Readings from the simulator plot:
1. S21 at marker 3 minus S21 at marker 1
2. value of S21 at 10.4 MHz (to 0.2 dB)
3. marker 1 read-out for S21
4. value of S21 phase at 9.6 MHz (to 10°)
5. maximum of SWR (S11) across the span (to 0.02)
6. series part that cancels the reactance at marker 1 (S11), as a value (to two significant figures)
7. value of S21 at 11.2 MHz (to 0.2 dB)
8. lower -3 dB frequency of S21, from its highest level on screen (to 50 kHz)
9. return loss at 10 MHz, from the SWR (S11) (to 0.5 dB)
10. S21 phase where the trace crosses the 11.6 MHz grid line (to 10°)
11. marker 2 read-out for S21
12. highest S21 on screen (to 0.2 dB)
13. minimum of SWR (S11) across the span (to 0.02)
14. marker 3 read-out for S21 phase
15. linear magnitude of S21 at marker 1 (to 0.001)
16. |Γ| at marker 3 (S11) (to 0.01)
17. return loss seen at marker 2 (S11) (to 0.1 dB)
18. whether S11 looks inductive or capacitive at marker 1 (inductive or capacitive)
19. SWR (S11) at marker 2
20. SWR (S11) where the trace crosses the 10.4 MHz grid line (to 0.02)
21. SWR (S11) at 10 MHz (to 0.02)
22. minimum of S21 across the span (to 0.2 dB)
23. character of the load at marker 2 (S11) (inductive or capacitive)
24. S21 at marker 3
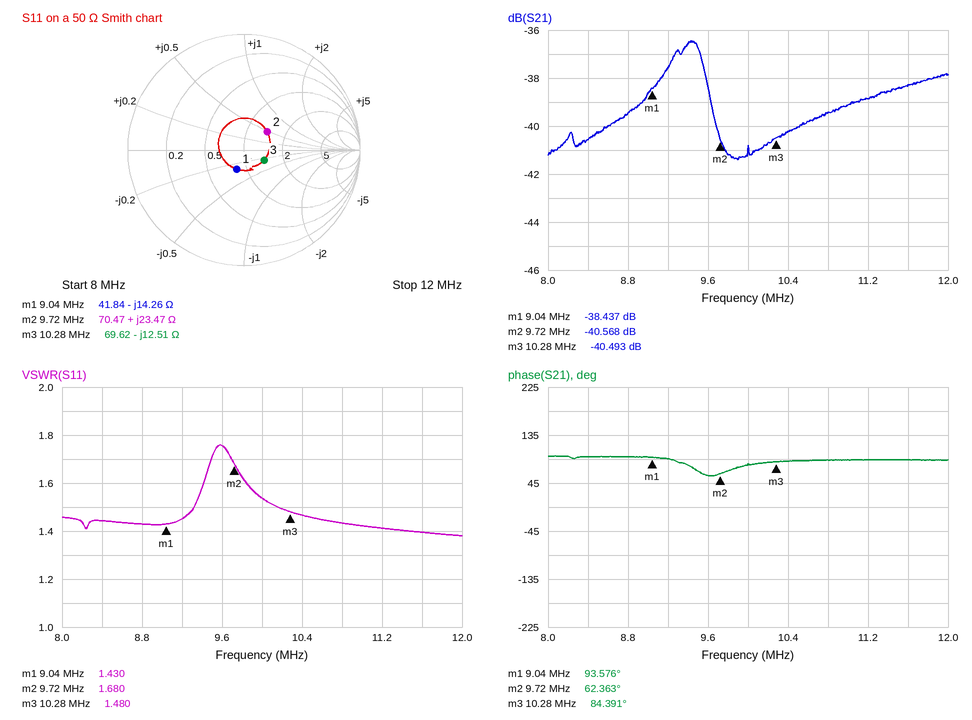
-2.056 dB
-40.2 dB
-38.437 dB
60°
1.76
250 nH
-38.8 dB
8.80 MHz
13.5 dB
90°
-40.568 dB
-36.4 dB
1.38
84.391°
0.012
0.19
11.9 dB
capacitive
1.680
1.46
1.54
-41.4 dB
inductive
-40.493 dB
